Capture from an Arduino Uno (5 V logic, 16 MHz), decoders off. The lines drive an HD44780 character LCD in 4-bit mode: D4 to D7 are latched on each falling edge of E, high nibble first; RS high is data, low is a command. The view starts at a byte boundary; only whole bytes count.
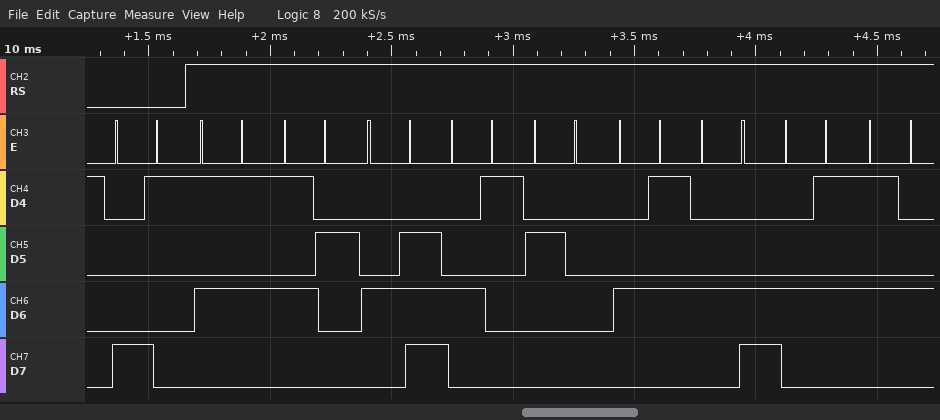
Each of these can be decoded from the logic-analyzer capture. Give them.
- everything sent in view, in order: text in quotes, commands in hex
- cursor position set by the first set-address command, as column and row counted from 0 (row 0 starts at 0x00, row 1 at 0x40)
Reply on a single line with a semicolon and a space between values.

0x81 "URNA ELET"; column 1, row 0
